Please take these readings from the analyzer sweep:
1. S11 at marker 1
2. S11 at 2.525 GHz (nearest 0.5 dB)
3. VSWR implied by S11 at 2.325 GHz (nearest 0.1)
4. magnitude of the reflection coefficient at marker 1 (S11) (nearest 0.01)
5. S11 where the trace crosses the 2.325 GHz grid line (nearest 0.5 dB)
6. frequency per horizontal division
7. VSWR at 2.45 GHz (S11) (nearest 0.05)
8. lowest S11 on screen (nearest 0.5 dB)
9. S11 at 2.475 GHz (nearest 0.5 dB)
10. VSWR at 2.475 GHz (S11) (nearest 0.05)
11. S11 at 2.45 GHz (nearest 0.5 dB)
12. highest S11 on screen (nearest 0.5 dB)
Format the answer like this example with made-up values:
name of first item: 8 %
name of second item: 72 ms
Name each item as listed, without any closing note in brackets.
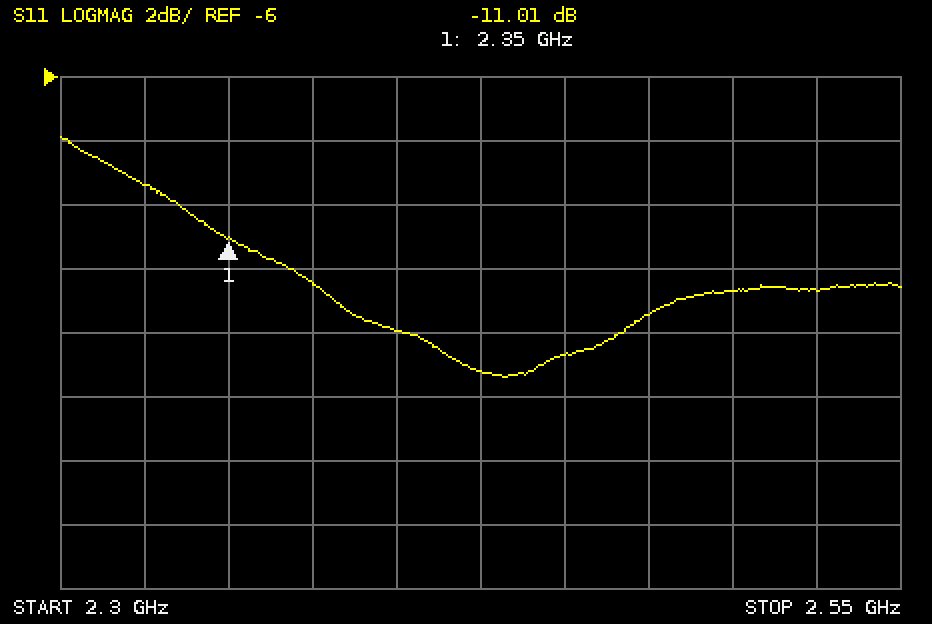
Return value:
S11 at marker 1: -11.01 dB
S11 at 2.525 GHz: -12.5 dB
VSWR implied by S11 at 2.325 GHz: 2.0
magnitude of the reflection coefficient at marker 1 (S11): 0.28
S11 where the trace crosses the 2.325 GHz grid line: -9.5 dB
frequency per horizontal division: 25 MHz
VSWR at 2.45 GHz (S11): 1.45
lowest S11 on screen: -15.5 dB
S11 at 2.475 GHz: -13.5 dB
VSWR at 2.475 GHz (S11): 1.55
S11 at 2.45 GHz: -14.5 dB
highest S11 on screen: -8.0 dB
